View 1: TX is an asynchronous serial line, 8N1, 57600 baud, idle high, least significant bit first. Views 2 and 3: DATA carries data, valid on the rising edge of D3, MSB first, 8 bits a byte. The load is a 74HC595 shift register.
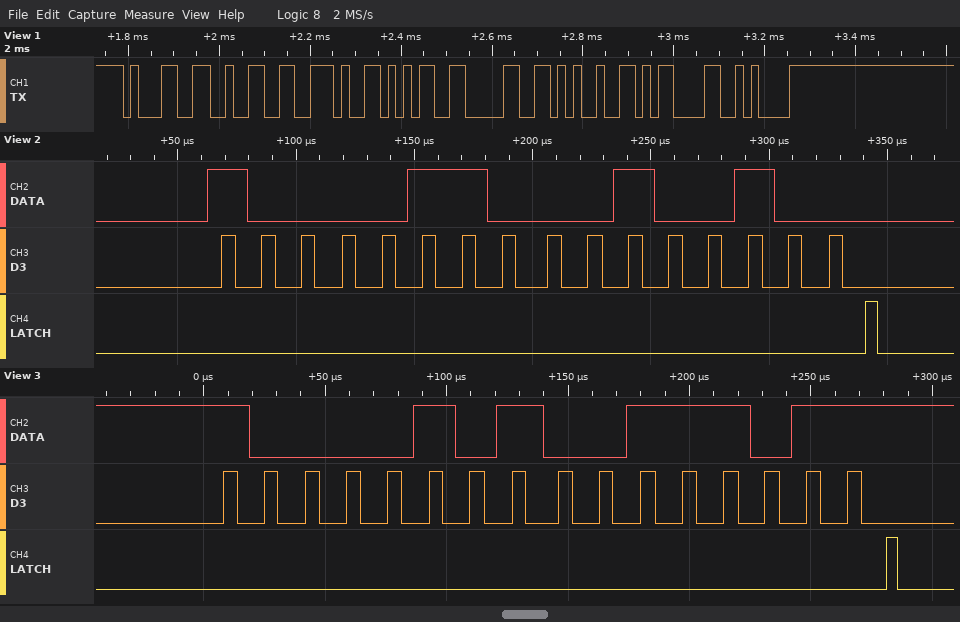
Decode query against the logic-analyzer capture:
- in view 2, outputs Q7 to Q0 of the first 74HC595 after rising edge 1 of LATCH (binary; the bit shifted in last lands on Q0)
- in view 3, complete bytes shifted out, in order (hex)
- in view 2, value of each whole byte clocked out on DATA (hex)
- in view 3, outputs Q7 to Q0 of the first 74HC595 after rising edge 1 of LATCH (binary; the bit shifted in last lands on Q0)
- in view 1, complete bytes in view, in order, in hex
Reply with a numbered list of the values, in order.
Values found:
1. 00100100
2. 0x85 0x3B
3. 86 24
4. 00111011
5. 31 32 2E 35 30 25 0D 0A
